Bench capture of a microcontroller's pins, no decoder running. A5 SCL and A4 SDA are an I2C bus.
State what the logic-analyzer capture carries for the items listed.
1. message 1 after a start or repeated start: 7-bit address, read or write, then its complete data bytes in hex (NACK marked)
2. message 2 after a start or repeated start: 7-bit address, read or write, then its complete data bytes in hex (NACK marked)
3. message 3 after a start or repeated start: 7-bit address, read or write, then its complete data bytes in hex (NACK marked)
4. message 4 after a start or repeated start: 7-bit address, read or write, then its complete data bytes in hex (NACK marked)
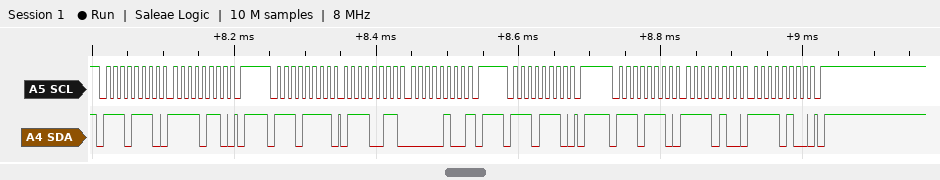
0x77 write: F6
0x77 read: 73 04 NACK
0x77 write
0x77 write: F4 F4
